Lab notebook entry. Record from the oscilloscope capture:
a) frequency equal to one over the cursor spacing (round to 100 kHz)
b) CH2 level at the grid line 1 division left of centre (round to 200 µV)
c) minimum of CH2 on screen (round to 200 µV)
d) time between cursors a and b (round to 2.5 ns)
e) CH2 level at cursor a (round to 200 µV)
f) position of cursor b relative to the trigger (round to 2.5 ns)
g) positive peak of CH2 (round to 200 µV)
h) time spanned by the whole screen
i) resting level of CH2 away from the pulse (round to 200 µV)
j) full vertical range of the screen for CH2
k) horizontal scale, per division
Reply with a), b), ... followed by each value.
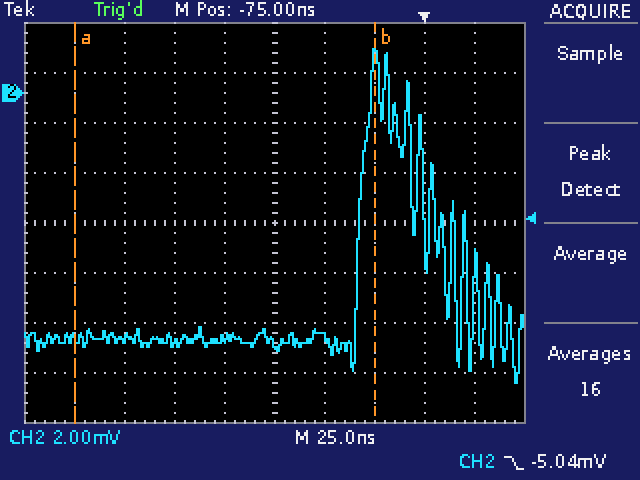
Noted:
a) 6.7 MHz
b) -9.8 mV
c) -11.6 mV
d) 150.0 ns
e) -9.8 mV
f) -25.0 ns
g) 1.8 mV
h) 250 ns
i) -9.8 mV
j) 16 mV
k) 25 ns
